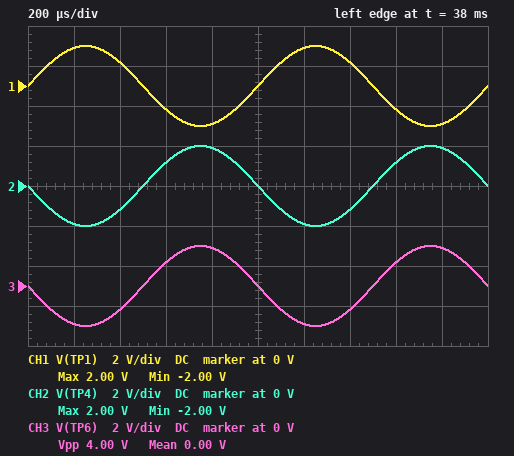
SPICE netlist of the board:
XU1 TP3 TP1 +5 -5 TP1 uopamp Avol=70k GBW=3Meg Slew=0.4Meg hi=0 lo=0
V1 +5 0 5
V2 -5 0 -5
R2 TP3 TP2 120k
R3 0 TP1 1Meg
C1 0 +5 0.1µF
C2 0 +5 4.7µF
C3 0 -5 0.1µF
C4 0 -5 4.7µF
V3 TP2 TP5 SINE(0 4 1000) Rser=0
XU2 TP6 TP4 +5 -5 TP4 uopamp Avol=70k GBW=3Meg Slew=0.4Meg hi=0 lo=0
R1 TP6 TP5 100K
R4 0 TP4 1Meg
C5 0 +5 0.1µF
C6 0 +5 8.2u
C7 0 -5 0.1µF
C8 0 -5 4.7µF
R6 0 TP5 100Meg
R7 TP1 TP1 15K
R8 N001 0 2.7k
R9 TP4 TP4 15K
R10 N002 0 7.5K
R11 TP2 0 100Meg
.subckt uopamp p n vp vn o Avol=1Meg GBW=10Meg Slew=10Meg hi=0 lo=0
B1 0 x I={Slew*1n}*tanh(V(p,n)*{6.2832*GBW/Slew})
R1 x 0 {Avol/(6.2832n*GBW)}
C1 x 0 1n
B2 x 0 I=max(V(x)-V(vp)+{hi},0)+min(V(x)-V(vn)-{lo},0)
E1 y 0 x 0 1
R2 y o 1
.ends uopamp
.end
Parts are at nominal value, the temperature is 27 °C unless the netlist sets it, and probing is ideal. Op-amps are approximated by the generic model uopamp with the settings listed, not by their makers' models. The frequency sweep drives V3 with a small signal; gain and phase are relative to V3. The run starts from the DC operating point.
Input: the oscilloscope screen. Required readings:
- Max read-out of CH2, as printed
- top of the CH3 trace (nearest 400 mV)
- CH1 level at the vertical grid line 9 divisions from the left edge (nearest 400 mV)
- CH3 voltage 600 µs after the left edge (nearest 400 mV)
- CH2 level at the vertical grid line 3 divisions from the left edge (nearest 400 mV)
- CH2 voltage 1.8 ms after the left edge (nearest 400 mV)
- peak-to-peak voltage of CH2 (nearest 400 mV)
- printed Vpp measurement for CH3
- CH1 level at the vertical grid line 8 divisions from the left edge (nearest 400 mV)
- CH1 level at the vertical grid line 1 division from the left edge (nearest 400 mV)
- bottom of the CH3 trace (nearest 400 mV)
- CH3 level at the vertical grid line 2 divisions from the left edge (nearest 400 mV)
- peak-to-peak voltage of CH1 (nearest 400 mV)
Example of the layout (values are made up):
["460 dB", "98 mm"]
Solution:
["2.00 V", "2.0 V", "-2.0 V", "1.2 V", "1.2 V", "2.0 V", "4.0 V", "4.00 V", "-1.2 V", "2.0 V", "-2.0 V", "-1.2 V", "4.0 V"]
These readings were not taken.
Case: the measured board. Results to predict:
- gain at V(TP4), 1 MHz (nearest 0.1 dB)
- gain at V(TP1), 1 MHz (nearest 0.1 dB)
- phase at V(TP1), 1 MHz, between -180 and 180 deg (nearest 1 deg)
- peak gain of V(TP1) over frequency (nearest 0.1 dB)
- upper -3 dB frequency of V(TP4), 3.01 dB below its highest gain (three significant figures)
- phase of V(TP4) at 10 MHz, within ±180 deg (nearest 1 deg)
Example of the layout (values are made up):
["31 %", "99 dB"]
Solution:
["-6.5 dB", "-6.5 dB", "-18 deg", "-6.0 dB", "3.00 MHz", "107 deg"]
